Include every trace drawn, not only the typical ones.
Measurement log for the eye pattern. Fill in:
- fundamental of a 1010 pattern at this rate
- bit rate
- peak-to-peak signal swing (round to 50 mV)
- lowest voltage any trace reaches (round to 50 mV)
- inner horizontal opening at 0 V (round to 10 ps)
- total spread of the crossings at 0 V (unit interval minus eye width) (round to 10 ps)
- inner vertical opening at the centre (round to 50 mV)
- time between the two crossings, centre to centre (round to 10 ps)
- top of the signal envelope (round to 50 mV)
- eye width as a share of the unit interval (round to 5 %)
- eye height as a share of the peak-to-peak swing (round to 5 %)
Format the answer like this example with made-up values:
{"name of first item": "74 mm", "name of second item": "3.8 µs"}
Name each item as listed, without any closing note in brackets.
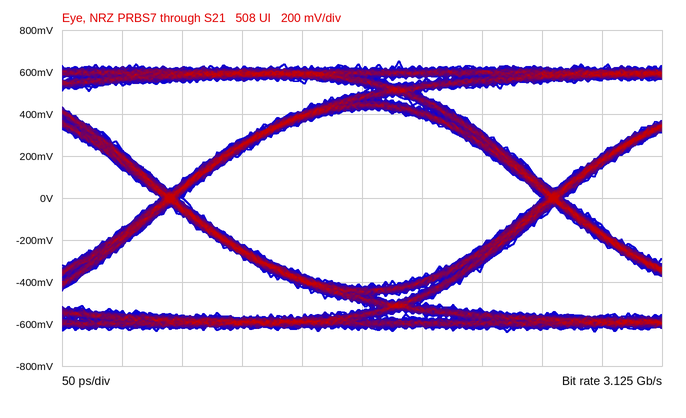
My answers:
{"fundamental of a 1010 pattern at this rate": "1.5625 GHz", "bit rate": "3.125 Gb/s", "peak-to-peak signal swing": "1.30 V", "lowest voltage any trace reaches": "-650 mV", "inner horizontal opening at 0 V": "300 ps", "total spread of the crossings at 0 V (unit interval minus eye width)": "20 ps", "inner vertical opening at the centre": "850 mV", "time between the two crossings, centre to centre": "320 ps", "top of the signal envelope": "650 mV", "eye width as a share of the unit interval": "95 %", "eye height as a share of the peak-to-peak swing": "65 %"}
